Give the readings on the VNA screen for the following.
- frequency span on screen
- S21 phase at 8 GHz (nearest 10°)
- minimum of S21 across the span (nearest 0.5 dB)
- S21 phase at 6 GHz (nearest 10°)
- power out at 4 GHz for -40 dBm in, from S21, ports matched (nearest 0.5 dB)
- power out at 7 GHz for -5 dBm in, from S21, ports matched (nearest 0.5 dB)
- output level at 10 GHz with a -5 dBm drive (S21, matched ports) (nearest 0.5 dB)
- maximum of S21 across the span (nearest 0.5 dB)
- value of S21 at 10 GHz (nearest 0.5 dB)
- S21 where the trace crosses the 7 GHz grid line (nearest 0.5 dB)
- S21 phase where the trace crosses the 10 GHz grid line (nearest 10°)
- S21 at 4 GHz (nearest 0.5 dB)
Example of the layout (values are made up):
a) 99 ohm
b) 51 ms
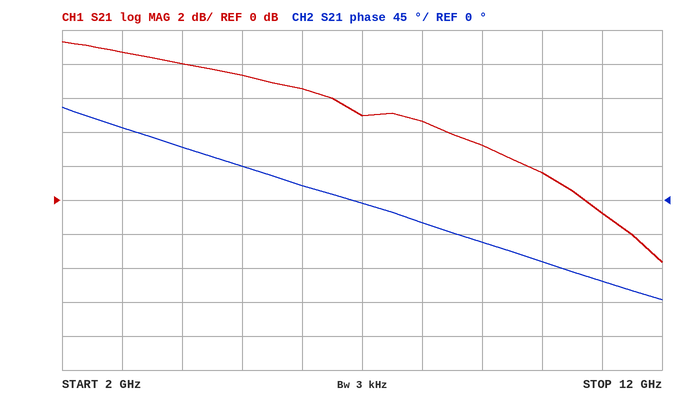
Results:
a) 10 GHz
b) -30°
c) -3.5 dB
d) 20°
e) -32.0 dBm
f) 0.0 dBm
g) -3.5 dBm
h) 9.5 dB
i) 1.5 dB
j) 5.0 dB
k) -80°
l) 8.0 dB
